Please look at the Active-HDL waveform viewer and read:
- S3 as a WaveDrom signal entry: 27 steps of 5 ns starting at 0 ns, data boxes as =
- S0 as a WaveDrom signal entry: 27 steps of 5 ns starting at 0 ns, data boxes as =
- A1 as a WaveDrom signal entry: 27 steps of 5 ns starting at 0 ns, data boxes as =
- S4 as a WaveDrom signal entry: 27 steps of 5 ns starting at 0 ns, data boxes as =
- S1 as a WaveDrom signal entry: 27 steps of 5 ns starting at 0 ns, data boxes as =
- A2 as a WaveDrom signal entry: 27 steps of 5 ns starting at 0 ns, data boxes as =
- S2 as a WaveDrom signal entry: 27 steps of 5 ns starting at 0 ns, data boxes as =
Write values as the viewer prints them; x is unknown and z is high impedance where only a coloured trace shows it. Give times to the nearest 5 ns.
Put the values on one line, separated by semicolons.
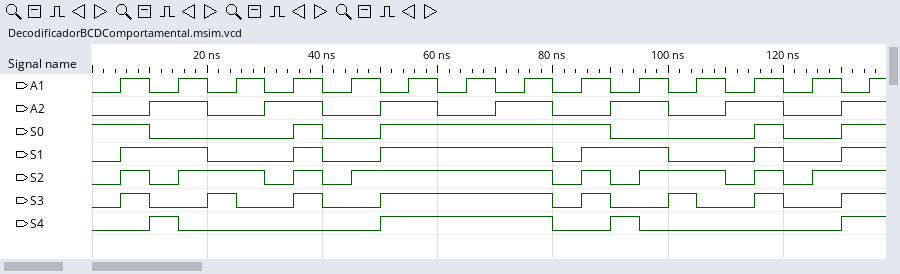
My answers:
{name: 'S3', wave: '010.10.10.1.....010.10.10.1'}; {name: 'S0', wave: '1.0....10.1.......0....10.1'}; {name: 'A1', wave: '010101010101010101010101010'}; {name: 'S4', wave: '0.10......1.....0.10......1'}; {name: 'S1', wave: '01..0..10.1.....01..0..10.1'}; {name: 'A2', wave: '0.1.0.1.0.1.0.1.0.1.0.1.0.1'}; {name: 'S2', wave: '0101..0101......0101..0101.'}
